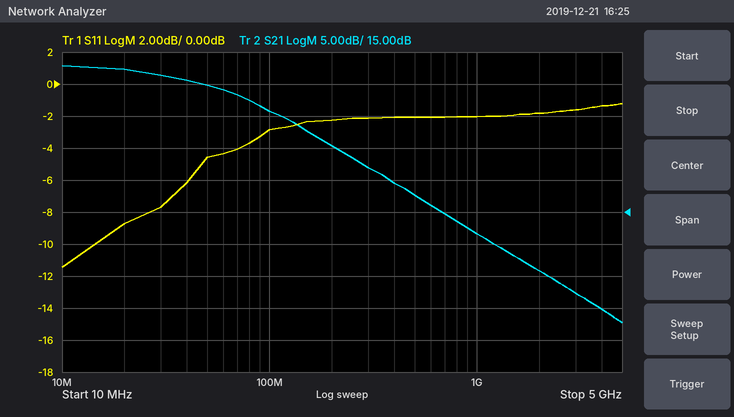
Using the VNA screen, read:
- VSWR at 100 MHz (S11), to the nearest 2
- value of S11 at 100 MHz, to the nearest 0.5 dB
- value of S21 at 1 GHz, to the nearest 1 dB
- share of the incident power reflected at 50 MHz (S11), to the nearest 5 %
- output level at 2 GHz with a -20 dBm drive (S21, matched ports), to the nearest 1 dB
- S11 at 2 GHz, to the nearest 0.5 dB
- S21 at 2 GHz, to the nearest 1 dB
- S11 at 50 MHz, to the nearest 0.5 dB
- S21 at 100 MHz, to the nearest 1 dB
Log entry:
6
-3.0 dB
12 dB
35 %
-14 dBm
-2.0 dB
6 dB
-4.5 dB
31 dB
